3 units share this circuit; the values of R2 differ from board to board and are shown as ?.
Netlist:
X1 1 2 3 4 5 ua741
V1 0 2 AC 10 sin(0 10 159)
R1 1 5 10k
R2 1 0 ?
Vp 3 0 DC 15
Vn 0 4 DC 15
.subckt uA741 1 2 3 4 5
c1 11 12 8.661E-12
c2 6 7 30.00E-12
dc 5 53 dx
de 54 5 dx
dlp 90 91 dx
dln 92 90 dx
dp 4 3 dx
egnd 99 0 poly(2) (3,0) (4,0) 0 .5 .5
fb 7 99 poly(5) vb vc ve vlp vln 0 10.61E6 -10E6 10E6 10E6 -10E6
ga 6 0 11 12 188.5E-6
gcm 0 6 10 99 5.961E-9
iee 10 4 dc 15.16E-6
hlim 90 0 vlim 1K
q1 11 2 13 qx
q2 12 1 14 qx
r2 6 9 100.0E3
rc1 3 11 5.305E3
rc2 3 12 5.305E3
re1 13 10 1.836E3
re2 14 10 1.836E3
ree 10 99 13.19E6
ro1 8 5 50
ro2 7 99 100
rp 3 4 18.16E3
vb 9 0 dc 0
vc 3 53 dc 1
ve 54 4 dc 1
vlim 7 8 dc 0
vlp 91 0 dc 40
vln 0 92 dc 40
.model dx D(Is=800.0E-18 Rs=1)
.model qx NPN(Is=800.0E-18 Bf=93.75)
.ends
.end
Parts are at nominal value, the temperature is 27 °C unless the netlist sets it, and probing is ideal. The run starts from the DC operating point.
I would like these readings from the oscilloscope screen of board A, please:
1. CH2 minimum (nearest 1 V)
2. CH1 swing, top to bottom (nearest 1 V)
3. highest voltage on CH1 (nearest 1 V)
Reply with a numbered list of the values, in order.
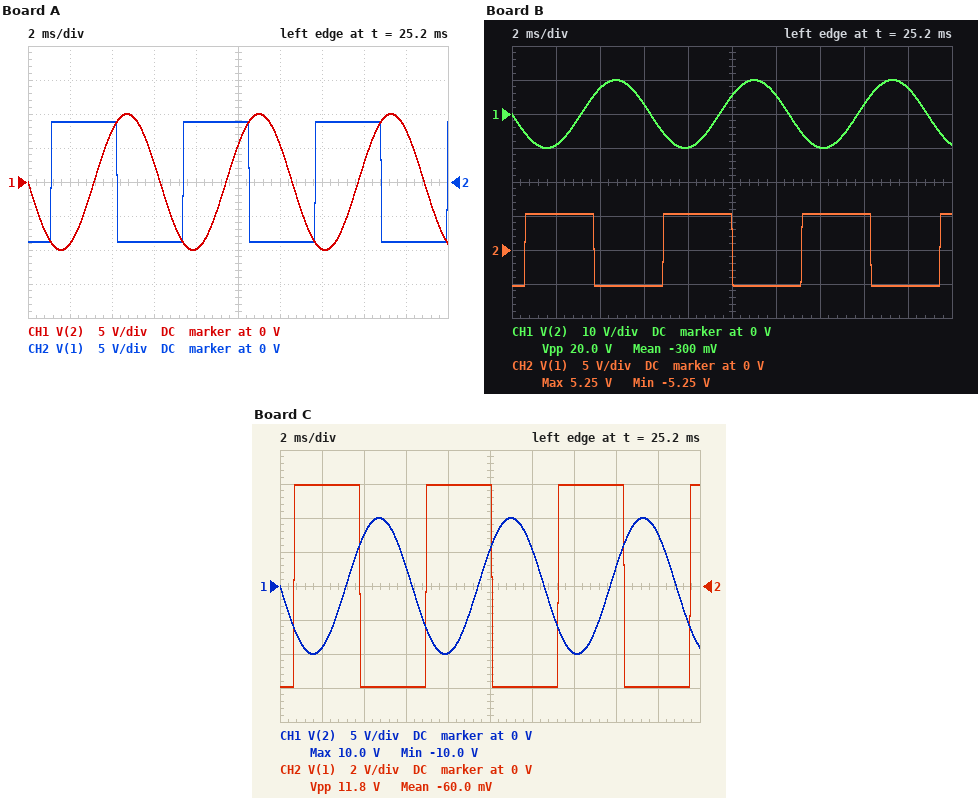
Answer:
1. -9 V
2. 20 V
3. 10 V
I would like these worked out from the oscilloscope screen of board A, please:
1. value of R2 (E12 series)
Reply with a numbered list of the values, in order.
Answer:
1. 15 kΩ
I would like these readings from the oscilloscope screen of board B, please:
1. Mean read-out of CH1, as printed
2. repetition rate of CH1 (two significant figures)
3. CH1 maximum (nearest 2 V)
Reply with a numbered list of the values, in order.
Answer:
1. -300 mV
2. 160 Hz
3. 10 V
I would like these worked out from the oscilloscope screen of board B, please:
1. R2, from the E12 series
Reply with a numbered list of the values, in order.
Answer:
1. 5.6 kΩ
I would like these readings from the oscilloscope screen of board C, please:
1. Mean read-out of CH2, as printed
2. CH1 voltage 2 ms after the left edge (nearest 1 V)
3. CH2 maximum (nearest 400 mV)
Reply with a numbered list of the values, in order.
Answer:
1. -60.0 mV
2. -9 V
3. 6.0 V
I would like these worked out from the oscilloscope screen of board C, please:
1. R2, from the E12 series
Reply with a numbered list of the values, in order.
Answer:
1. 6.8 kΩ
